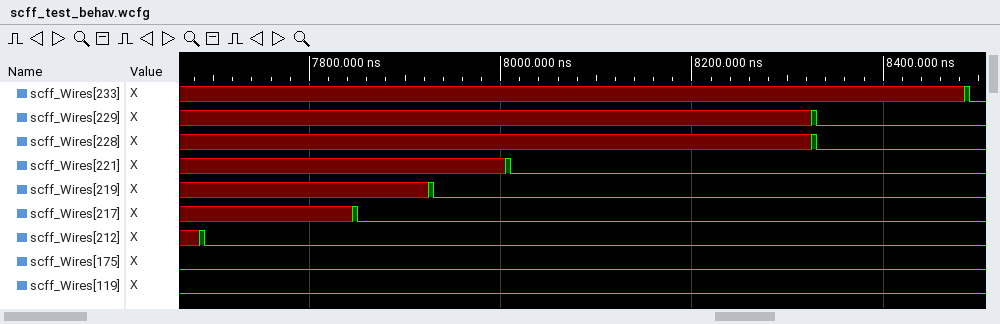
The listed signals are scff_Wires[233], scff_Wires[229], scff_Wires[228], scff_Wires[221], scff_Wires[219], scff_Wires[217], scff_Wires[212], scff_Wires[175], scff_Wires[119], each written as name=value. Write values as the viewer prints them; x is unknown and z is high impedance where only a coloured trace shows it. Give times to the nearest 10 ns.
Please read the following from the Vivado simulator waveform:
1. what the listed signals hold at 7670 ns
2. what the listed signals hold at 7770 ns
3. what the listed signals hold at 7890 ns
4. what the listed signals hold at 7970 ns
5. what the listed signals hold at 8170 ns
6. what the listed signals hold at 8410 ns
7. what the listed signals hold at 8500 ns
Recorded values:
scff_Wires[233]=x, scff_Wires[229]=x, scff_Wires[228]=x, scff_Wires[221]=x, scff_Wires[219]=x, scff_Wires[217]=x, scff_Wires[212]=x, scff_Wires[175]=0, scff_Wires[119]=0
scff_Wires[233]=x, scff_Wires[229]=x, scff_Wires[228]=x, scff_Wires[221]=x, scff_Wires[219]=x, scff_Wires[217]=x, scff_Wires[212]=0, scff_Wires[175]=0, scff_Wires[119]=0
scff_Wires[233]=x, scff_Wires[229]=x, scff_Wires[228]=x, scff_Wires[221]=x, scff_Wires[219]=x, scff_Wires[217]=0, scff_Wires[212]=0, scff_Wires[175]=0, scff_Wires[119]=0
scff_Wires[233]=x, scff_Wires[229]=x, scff_Wires[228]=x, scff_Wires[221]=x, scff_Wires[219]=0, scff_Wires[217]=0, scff_Wires[212]=0, scff_Wires[175]=0, scff_Wires[119]=0
scff_Wires[233]=x, scff_Wires[229]=x, scff_Wires[228]=x, scff_Wires[221]=0, scff_Wires[219]=0, scff_Wires[217]=0, scff_Wires[212]=0, scff_Wires[175]=0, scff_Wires[119]=0
scff_Wires[233]=x, scff_Wires[229]=0, scff_Wires[228]=0, scff_Wires[221]=0, scff_Wires[219]=0, scff_Wires[217]=0, scff_Wires[212]=0, scff_Wires[175]=0, scff_Wires[119]=0
scff_Wires[233]=0, scff_Wires[229]=0, scff_Wires[228]=0, scff_Wires[221]=0, scff_Wires[219]=0, scff_Wires[217]=0, scff_Wires[212]=0, scff_Wires[175]=0, scff_Wires[119]=0
